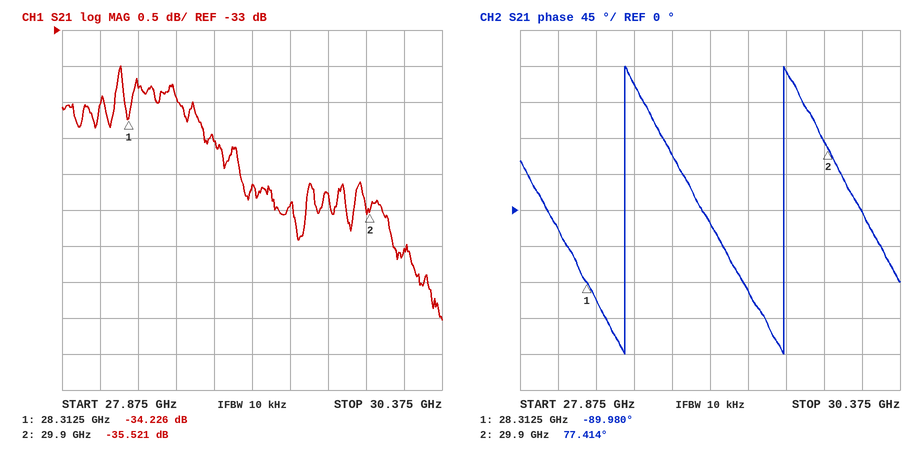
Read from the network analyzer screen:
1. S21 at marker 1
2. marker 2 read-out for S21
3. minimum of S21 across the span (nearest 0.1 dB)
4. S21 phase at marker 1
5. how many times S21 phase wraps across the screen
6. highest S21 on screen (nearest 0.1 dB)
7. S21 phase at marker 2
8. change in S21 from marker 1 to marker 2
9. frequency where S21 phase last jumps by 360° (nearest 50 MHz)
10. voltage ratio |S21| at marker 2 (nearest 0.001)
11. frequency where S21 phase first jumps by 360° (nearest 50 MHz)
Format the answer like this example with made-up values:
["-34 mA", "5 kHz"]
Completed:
["-34.226 dB", "-35.521 dB", "-37.0 dB", "-89.980°", "2", "-33.5 dB", "77.414°", "-1.295 dB", "29.60 GHz", "0.017", "28.55 GHz"]
